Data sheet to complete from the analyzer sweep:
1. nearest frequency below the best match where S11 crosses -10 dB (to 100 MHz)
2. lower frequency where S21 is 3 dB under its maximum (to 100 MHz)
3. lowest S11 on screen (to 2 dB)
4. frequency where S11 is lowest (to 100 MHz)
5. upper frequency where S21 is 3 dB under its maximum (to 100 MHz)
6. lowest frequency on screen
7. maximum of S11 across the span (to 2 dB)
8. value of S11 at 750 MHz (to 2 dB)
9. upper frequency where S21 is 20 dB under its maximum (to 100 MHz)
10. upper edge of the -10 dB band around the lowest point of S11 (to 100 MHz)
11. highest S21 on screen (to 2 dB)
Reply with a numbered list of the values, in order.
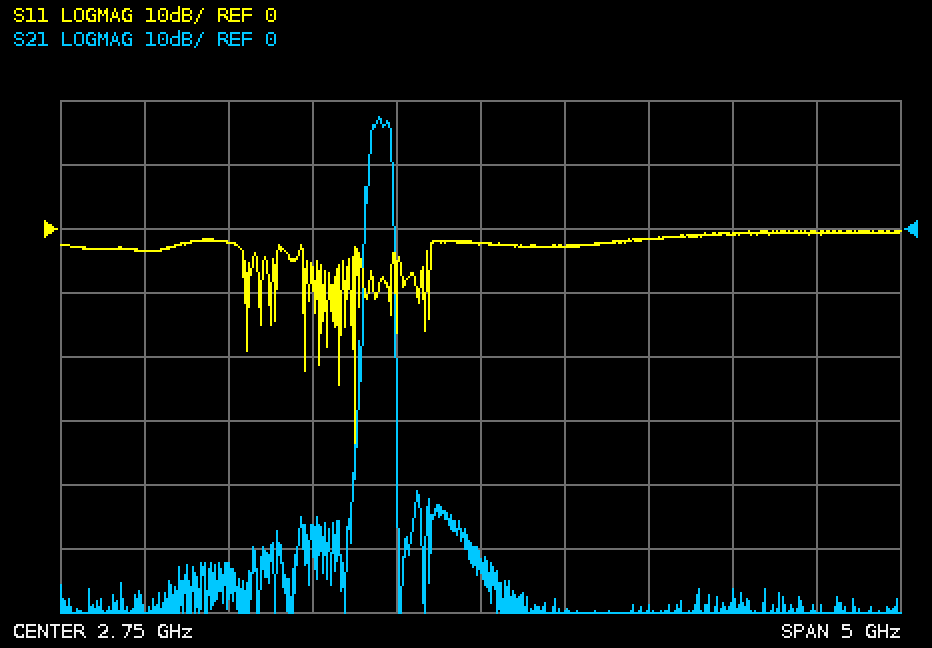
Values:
1. 2.0 GHz
2. 2.1 GHz
3. -34 dB
4. 2.0 GHz
5. 2.2 GHz
6. 250 MHz
7. 0 dB
8. -4 dB
9. 2.2 GHz
10. 2.0 GHz
11. 18 dB
